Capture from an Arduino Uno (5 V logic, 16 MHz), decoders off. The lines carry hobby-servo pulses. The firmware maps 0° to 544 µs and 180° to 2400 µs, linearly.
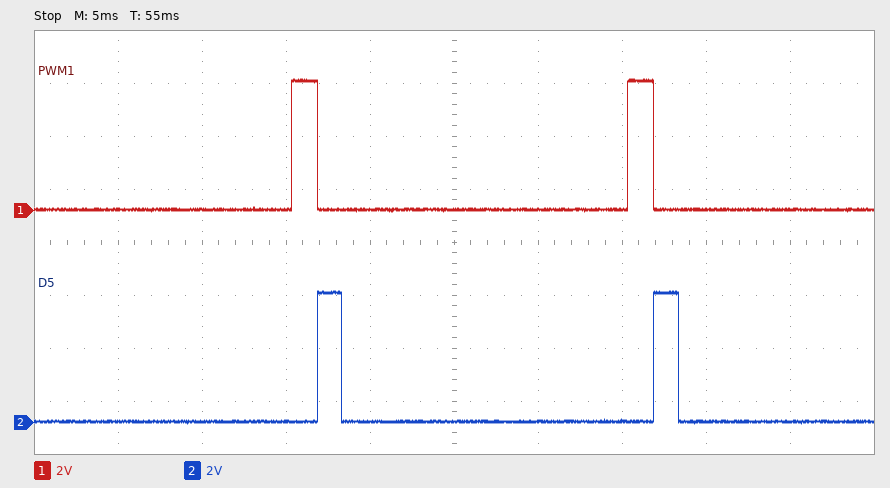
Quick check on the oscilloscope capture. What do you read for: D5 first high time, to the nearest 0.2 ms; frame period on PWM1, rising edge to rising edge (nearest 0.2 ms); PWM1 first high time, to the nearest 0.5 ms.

1.4 ms
20.0 ms
1.5 ms
